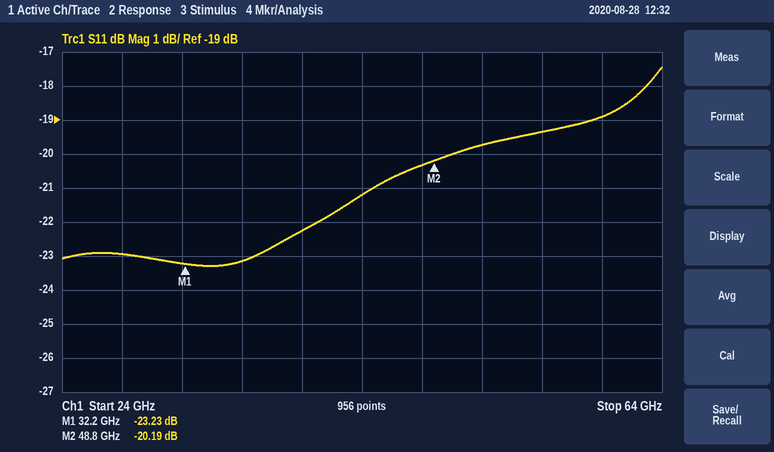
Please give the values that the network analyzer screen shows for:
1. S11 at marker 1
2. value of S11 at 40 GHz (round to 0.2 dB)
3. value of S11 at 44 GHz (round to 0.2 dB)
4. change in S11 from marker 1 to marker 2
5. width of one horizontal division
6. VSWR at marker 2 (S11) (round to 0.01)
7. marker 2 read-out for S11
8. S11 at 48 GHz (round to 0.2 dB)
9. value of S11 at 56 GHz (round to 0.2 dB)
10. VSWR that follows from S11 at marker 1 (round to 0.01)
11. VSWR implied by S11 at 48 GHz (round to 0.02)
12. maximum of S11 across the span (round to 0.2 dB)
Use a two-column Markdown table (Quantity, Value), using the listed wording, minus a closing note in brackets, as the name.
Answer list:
| Quantity | Value |
|---|---|
| S11 at marker 1 | -23.23 dB |
| value of S11 at 40 GHz | -22.2 dB |
| value of S11 at 44 GHz | -21.2 dB |
| change in S11 from marker 1 to marker 2 | 3.04 dB |
| width of one horizontal division | 4 GHz |
| VSWR at marker 2 (S11) | 1.22 |
| marker 2 read-out for S11 | -20.19 dB |
| S11 at 48 GHz | -20.4 dB |
| value of S11 at 56 GHz | -19.4 dB |
| VSWR that follows from S11 at marker 1 | 1.15 |
| VSWR implied by S11 at 48 GHz | 1.22 |
| maximum of S11 across the span | -17.4 dB |
